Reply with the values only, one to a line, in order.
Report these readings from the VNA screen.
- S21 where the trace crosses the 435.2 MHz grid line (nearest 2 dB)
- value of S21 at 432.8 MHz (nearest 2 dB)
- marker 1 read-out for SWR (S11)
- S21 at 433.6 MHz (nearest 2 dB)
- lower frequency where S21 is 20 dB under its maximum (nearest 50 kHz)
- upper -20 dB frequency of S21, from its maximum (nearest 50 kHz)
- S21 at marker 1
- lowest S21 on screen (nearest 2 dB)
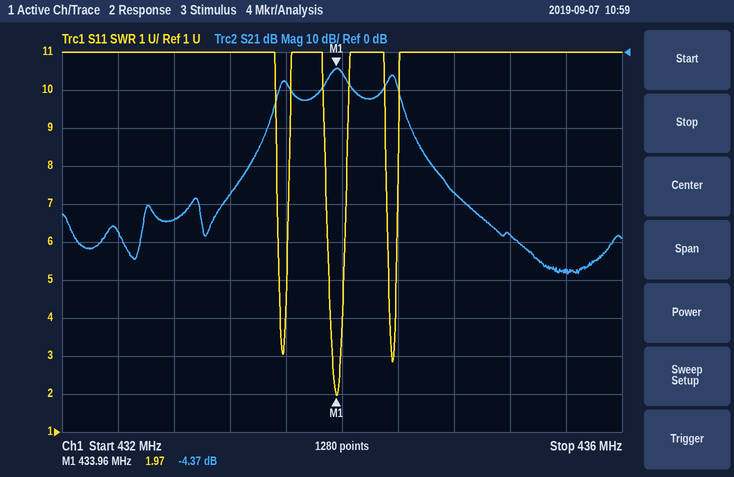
-48 dB
-44 dB
1.97
-8 dB
433.40 MHz
434.55 MHz
-4.37 dB
-58 dB
